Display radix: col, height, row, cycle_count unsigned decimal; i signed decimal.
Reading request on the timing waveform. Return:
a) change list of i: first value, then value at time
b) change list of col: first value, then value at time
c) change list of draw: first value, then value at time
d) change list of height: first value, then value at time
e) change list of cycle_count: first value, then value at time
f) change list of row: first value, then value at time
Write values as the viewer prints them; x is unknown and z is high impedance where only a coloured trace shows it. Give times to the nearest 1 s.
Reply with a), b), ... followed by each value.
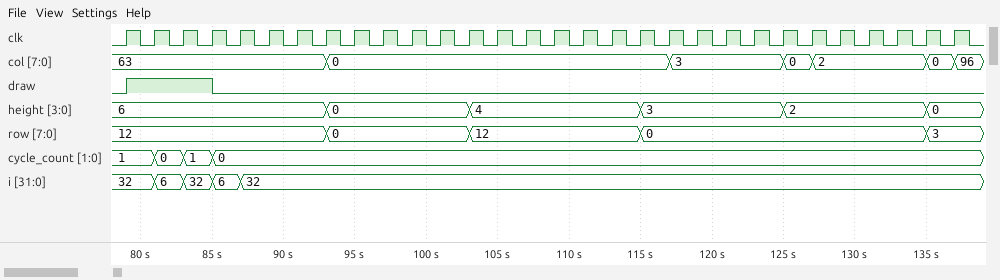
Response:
a) 32, 6 at 81 s, 32 at 83 s, 6 at 85 s, 32 at 87 s
b) 63, 0 at 93 s, 3 at 117 s, 0 at 125 s, 2 at 127 s, 0 at 135 s, 96 at 137 s
c) 0, 1 at 79 s, 0 at 85 s
d) 6, 0 at 93 s, 4 at 103 s, 3 at 115 s, 2 at 125 s, 0 at 135 s
e) 1, 0 at 81 s, 1 at 83 s, 0 at 85 s
f) 12, 0 at 93 s, 12 at 103 s, 0 at 115 s, 3 at 135 s
